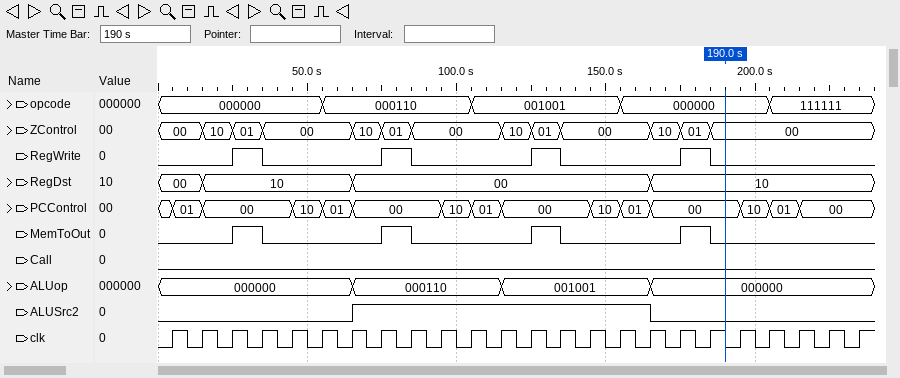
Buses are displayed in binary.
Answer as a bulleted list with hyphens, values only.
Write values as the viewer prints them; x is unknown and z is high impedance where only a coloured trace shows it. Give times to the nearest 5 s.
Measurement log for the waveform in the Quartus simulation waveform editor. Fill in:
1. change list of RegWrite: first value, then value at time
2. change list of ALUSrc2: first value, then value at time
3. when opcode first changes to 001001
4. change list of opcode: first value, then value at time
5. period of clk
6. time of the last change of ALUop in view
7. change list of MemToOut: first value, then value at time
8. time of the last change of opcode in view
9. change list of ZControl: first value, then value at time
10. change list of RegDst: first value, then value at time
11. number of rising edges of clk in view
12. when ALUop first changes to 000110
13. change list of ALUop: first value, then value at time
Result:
- 0, 1 at 25 s, 0 at 35 s, 1 at 75 s, 0 at 85 s, 1 at 125 s, 0 at 135 s, 1 at 175 s, 0 at 185 s
- 0, 1 at 65 s, 0 at 165 s
- 105 s
- 000000, 000110 at 55 s, 001001 at 105 s, 000000 at 155 s, 111111 at 205 s
- 10 s
- 165 s
- 0, 1 at 25 s, 0 at 35 s, 1 at 75 s, 0 at 85 s, 1 at 125 s, 0 at 135 s, 1 at 175 s, 0 at 185 s
- 205 s
- 00, 10 at 15 s, 01 at 25 s, 00 at 35 s, 10 at 65 s, 01 at 75 s, 00 at 85 s, 10 at 115 s, 01 at 125 s, 00 at 135 s, 10 at 165 s, 01 at 175 s, 00 at 185 s
- 00, 10 at 15 s, 00 at 65 s, 10 at 165 s
- 24
- 65 s
- 000000, 000110 at 65 s, 001001 at 115 s, 000000 at 165 s
